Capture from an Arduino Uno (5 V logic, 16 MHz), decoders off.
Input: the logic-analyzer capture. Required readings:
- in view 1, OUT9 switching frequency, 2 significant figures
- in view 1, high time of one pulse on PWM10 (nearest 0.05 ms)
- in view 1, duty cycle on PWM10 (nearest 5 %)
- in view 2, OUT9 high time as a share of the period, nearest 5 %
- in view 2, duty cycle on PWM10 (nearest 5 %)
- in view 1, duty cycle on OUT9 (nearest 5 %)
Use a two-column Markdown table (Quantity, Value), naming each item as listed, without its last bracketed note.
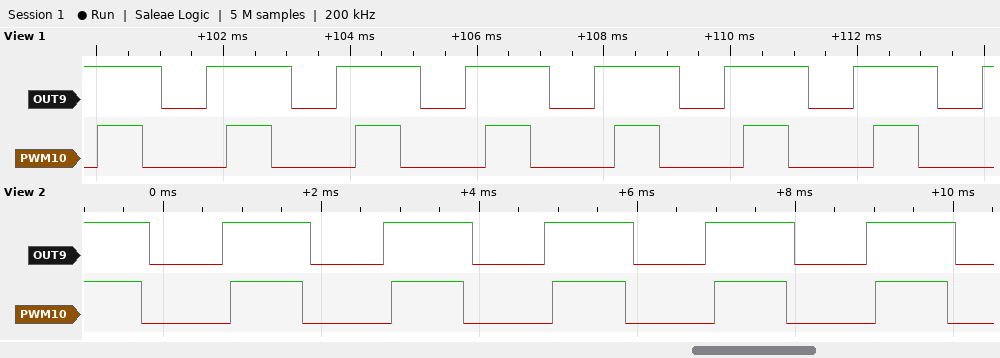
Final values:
| Quantity | Value |
|---|---|
| in view 1, OUT9 switching frequency, 2 significant figures | 490 Hz |
| in view 1, high time of one pulse on PWM10 | 0.70 ms |
| in view 1, duty cycle on PWM10 | 35 % |
| in view 2, OUT9 high time as a share of the period, nearest 5 % | 55 % |
| in view 2, duty cycle on PWM10 | 45 % |
| in view 1, duty cycle on OUT9 | 65 % |
